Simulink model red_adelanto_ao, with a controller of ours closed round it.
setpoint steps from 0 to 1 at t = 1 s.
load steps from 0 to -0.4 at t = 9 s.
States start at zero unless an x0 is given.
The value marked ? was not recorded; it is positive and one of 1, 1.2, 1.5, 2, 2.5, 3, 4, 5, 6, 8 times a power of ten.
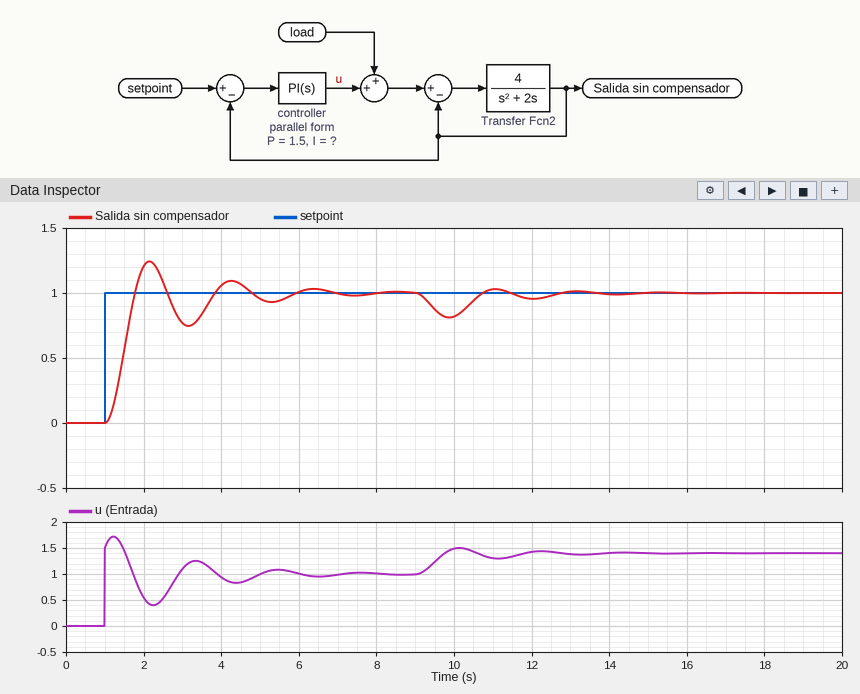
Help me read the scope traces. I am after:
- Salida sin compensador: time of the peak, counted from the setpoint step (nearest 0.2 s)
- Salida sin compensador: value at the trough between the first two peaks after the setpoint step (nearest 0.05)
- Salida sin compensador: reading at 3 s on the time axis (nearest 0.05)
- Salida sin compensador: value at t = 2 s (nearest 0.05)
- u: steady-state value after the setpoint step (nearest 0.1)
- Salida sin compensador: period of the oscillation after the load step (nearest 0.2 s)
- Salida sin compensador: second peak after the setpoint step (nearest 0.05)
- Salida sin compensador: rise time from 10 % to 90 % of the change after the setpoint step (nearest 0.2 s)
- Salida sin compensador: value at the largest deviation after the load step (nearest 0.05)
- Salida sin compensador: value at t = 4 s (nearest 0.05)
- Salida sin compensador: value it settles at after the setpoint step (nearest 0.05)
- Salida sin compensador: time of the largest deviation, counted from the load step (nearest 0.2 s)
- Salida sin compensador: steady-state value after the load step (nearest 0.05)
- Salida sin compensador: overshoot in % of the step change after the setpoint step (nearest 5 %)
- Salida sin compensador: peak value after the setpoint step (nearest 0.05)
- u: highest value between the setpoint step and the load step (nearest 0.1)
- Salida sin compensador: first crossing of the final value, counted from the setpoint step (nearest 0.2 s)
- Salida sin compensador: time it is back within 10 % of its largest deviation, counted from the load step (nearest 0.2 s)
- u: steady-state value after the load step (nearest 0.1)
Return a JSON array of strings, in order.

["1.2 s", "0.75", "0.75", "1.20", "1.0", "2.2 s", "1.10", "0.6 s", "0.80", "1.05", "1.00", "0.8 s", "1.00", "25 %", "1.25", "1.7", "0.8 s", "3.6 s", "1.4"]
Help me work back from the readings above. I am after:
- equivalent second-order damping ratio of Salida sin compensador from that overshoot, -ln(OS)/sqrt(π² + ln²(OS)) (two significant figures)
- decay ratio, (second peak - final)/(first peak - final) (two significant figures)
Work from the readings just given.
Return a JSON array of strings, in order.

["0.40", "0.40"]
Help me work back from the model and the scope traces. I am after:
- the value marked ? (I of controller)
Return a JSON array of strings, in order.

["2"]
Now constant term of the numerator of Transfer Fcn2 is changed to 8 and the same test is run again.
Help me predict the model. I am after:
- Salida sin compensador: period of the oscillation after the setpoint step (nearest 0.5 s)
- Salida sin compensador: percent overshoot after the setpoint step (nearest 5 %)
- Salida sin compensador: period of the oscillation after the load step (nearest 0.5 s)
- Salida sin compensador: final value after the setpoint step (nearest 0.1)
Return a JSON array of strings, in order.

["1.5 s", "20 %", "1.5 s", "1.0"]
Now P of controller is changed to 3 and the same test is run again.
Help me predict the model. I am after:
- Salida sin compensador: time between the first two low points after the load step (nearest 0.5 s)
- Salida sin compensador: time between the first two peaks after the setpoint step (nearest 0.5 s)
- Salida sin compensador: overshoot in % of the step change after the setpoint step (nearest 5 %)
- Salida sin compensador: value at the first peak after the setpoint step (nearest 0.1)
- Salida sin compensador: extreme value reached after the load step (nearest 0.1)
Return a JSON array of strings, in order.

["1.5 s", "1.5 s", "30 %", "1.3", "0.9"]
